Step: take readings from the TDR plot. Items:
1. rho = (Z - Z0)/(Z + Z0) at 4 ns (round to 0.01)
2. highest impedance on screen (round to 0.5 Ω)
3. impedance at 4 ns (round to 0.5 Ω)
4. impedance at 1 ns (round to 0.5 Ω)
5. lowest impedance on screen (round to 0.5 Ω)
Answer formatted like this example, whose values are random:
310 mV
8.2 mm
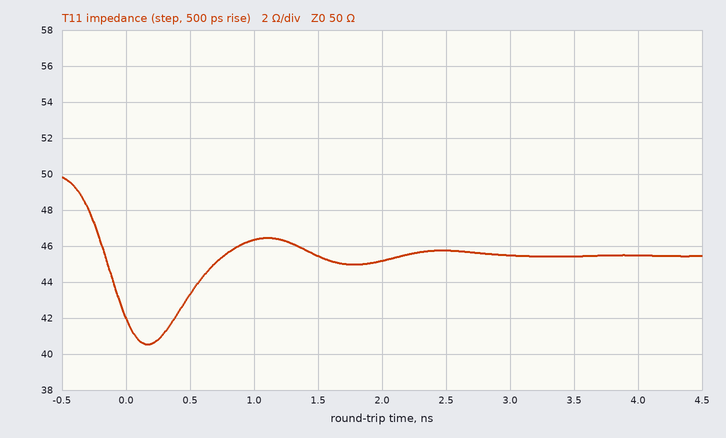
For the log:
-0.05
50.0 Ω
45.5 Ω
46.5 Ω
40.5 Ω
